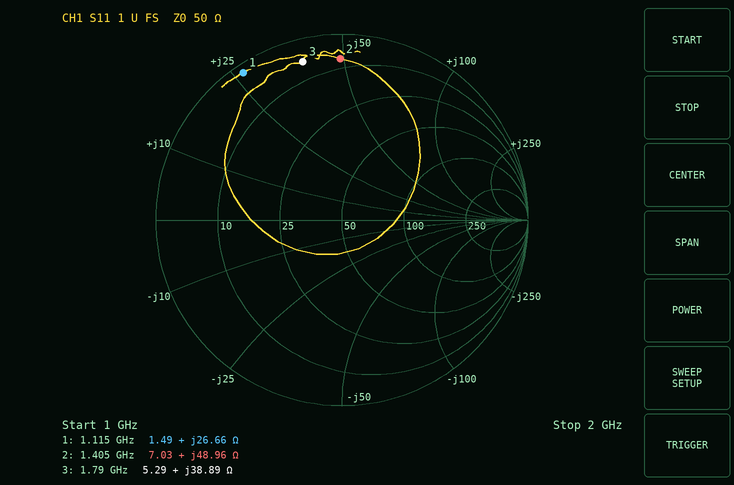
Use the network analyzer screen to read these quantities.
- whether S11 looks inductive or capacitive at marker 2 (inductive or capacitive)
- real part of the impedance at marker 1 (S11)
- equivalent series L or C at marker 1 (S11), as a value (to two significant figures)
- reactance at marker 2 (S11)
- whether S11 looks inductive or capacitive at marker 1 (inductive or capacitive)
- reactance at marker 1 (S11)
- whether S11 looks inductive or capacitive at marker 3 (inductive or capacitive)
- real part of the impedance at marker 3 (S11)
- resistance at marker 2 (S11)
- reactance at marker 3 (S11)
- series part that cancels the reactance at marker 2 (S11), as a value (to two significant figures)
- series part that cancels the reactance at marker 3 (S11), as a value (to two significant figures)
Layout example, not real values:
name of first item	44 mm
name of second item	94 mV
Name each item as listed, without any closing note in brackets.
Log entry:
whether S11 looks inductive or capacitive at marker 2	inductive
real part of the impedance at marker 1	1.49 Ω
equivalent series L or C at marker 1 (S11), as a value	3.8 nH
reactance at marker 2	+48.96 Ω
whether S11 looks inductive or capacitive at marker 1	inductive
reactance at marker 1	+26.66 Ω
whether S11 looks inductive or capacitive at marker 3	inductive
real part of the impedance at marker 3	5.29 Ω
resistance at marker 2	7.03 Ω
reactance at marker 3	+38.89 Ω
series part that cancels the reactance at marker 2 (S11), as a value	2.3 pF
series part that cancels the reactance at marker 3 (S11), as a value	2.3 pF
